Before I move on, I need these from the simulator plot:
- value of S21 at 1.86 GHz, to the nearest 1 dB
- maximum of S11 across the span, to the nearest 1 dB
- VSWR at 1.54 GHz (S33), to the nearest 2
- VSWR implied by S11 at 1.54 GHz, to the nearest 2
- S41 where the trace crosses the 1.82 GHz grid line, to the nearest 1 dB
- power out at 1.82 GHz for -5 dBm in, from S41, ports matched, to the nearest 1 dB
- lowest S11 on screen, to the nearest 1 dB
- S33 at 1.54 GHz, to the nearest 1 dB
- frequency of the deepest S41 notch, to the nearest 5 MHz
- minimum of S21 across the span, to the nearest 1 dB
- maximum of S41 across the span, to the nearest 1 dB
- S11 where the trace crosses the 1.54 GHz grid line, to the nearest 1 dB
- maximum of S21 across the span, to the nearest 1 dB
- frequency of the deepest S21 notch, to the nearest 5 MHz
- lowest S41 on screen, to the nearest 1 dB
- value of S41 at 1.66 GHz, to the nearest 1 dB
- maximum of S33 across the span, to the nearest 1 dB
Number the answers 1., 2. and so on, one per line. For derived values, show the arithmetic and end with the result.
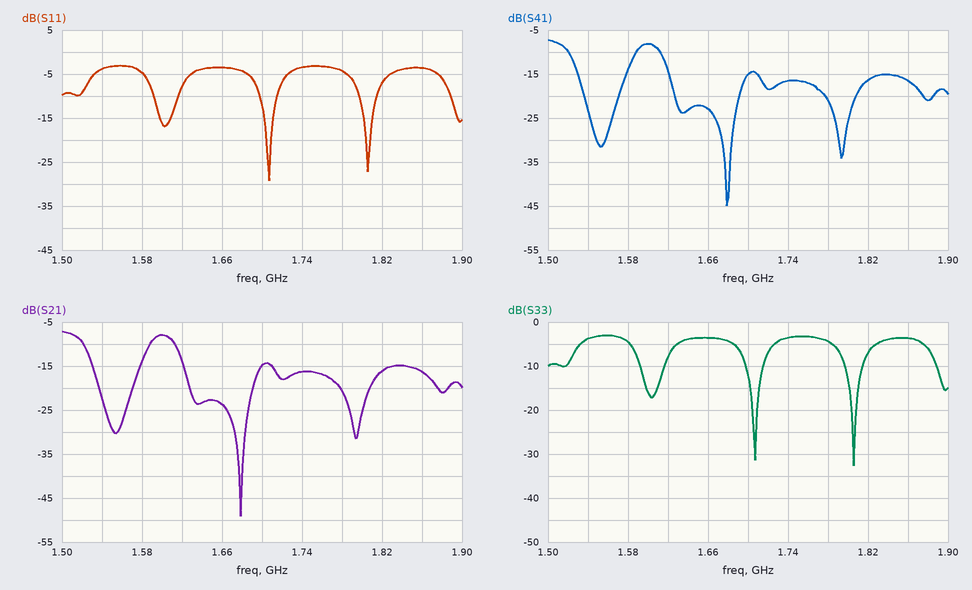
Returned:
1. -16 dB
2. -3 dB
3. |Γ| = 10^(-4/20) = 0.6310; VSWR = (1 + 0.6310)/(1 − 0.6310) ≈ 4
4. |Γ| = 10^(-4/20) = 0.6310; VSWR = (1 + 0.6310)/(1 − 0.6310) ≈ 4
5. -16 dB
6. -5 dBm + (-16 dB) = -21 dBm
7. -29 dB
8. -4 dB
9. 1.680 GHz
10. -49 dB
11. -7 dB
12. -4 dB
13. -7 dB
14. 1.680 GHz
15. -45 dB
16. -23 dB
17. -3 dB
